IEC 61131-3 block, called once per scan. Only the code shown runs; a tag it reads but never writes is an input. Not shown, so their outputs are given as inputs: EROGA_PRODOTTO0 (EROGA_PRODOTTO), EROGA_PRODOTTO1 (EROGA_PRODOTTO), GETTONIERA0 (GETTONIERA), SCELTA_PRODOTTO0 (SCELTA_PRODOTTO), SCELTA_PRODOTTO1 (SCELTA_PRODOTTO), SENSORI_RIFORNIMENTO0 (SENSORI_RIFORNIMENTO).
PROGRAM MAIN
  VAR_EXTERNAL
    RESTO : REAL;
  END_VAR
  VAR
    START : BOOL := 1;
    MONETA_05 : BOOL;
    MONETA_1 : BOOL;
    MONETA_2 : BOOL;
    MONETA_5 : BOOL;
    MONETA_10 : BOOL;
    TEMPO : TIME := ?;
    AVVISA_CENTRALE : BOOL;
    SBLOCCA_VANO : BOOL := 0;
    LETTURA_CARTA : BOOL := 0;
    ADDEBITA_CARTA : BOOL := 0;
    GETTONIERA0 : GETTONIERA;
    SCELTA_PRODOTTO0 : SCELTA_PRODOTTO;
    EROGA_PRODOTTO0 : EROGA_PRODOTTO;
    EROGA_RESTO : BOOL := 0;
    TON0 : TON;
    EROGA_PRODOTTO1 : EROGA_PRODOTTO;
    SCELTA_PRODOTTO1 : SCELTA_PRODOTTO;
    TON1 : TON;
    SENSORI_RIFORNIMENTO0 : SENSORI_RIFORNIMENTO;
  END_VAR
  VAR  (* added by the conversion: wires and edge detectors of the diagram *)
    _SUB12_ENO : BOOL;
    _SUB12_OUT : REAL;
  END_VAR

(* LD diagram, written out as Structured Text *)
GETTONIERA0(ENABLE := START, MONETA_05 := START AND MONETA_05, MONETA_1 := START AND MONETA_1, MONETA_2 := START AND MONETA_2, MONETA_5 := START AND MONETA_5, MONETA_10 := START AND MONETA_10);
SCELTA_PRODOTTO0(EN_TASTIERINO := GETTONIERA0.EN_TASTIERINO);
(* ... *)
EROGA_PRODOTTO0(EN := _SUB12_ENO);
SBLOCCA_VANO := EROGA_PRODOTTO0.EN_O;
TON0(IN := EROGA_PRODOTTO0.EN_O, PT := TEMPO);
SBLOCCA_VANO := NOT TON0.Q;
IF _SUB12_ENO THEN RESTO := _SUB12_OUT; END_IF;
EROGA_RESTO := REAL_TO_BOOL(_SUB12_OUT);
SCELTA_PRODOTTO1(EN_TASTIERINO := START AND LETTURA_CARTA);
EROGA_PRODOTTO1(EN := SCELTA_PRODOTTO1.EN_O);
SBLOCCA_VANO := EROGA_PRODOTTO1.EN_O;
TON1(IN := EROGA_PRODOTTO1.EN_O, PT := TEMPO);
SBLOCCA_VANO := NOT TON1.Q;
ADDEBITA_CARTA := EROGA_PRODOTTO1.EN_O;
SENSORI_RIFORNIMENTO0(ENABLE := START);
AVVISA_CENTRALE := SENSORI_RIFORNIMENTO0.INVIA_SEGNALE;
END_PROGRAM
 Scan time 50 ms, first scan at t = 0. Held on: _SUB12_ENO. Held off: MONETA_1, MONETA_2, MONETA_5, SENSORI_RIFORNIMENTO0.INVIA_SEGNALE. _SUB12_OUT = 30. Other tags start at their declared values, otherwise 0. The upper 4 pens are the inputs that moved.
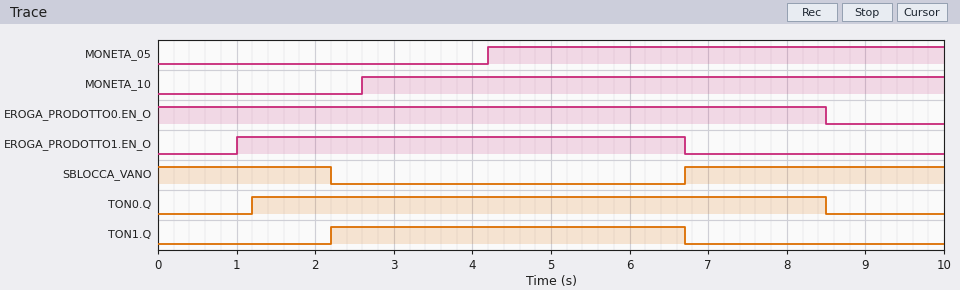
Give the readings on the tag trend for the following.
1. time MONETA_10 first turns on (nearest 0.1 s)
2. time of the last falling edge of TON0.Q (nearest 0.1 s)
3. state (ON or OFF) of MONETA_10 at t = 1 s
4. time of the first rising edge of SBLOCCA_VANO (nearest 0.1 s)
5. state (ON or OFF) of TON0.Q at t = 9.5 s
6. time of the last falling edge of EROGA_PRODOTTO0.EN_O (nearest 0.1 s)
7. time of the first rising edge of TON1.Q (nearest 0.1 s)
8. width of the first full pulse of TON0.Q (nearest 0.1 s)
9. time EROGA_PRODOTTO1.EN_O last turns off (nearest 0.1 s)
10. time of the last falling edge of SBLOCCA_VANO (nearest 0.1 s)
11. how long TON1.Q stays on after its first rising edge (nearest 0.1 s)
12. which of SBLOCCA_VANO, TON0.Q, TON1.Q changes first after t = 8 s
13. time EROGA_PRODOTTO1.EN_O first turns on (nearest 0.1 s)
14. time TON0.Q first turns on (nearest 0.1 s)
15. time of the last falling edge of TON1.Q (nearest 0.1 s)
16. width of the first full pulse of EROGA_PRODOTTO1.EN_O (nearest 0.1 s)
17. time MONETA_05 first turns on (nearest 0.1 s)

2.6 s
8.5 s
OFF
6.7 s
OFF
8.5 s
2.2 s
7.3 s
6.7 s
2.2 s
4.5 s
TON0.Q
1.0 s
1.2 s
6.7 s
5.7 s
4.2 s
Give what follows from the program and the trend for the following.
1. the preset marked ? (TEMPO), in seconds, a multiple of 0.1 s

1.2 s
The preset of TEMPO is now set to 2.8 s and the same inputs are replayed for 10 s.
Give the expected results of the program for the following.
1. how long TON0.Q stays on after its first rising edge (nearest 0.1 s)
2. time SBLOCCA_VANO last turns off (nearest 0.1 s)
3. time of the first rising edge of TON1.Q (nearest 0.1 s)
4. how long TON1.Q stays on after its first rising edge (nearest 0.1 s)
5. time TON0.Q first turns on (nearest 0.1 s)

5.7 s
3.8 s
3.8 s
2.9 s
2.8 s
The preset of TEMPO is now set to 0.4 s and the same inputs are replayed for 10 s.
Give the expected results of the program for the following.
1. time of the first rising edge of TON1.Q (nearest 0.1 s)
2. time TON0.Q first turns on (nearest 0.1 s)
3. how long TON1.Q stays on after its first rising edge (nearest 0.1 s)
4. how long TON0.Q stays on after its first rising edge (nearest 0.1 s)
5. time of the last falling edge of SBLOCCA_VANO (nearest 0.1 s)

1.4 s
0.4 s
5.3 s
8.1 s
1.4 s
